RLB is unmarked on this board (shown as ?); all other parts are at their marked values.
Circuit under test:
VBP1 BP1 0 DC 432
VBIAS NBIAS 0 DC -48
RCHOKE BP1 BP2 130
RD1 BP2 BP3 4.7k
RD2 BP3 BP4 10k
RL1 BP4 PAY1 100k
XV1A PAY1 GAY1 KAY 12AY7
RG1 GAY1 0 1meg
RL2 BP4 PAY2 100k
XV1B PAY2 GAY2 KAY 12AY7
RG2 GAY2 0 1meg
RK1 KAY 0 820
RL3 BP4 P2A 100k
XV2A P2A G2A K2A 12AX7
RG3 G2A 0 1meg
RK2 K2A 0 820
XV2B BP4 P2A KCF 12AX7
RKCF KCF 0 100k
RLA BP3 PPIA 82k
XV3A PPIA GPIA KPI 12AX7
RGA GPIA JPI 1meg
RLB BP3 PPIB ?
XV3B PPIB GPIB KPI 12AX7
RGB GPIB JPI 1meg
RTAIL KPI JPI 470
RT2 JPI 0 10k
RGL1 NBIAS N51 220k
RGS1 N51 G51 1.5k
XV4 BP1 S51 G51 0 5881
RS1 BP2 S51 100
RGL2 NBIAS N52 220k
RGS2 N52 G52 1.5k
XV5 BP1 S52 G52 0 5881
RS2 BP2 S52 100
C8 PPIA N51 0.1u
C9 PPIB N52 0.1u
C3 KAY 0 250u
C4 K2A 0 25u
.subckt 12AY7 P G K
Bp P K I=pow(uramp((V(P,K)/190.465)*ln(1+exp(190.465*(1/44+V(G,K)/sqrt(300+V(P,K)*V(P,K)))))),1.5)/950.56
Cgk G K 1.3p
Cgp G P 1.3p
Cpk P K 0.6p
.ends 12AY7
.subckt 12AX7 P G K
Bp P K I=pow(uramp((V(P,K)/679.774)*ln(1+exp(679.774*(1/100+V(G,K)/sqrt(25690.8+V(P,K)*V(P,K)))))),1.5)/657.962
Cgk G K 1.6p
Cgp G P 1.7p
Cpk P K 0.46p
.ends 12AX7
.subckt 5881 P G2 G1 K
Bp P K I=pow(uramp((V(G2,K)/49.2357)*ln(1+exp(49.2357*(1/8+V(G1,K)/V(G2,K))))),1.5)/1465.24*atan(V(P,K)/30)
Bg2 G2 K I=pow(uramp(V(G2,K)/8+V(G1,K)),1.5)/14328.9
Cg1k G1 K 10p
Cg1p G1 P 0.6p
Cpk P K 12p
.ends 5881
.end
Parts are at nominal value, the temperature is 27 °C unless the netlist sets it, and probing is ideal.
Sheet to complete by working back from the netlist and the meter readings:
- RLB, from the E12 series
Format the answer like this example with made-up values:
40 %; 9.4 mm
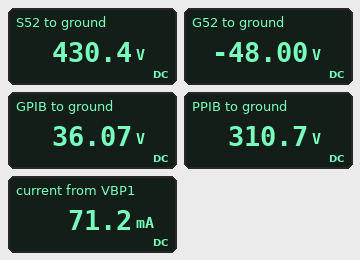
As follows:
33 kΩ
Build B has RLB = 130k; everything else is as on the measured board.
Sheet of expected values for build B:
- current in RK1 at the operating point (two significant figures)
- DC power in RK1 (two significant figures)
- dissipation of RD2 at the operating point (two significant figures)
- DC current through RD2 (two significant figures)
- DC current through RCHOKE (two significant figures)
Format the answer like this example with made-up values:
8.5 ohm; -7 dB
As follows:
3.2 mA; 8.2 mW; 410 mW; 6.4 mA; 11 mA
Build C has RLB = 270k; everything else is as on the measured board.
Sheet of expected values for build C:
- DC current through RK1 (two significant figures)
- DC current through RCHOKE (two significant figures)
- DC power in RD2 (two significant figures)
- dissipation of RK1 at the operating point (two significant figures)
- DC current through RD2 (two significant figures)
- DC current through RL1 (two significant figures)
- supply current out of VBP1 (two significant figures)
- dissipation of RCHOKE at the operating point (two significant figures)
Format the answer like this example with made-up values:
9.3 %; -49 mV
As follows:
3.2 mA; 11 mA; 410 mW; 8.3 mW; 6.4 mA; 1.6 mA; 70 mA; 16 mW
